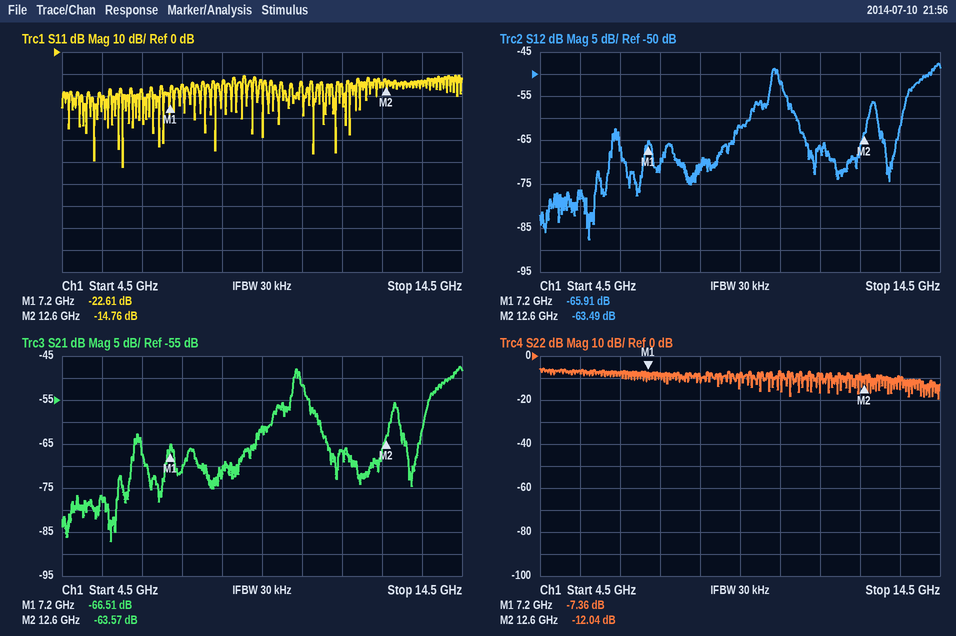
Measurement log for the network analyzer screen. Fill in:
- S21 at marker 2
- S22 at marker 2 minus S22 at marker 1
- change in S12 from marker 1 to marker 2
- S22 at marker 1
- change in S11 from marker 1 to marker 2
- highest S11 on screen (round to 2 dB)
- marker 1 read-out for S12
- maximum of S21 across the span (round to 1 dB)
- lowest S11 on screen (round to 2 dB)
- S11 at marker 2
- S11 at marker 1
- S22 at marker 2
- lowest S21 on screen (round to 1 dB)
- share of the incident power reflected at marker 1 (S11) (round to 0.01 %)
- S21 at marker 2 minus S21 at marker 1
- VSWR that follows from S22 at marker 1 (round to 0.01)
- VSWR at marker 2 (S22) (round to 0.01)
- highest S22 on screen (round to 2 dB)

-63.57 dB
-4.68 dB
2.42 dB
-7.36 dB
7.85 dB
-10 dB
-65.91 dB
-47 dB
-52 dB
-14.76 dB
-22.61 dB
-12.04 dB
-87 dB
0.55 %
2.94 dB
2.50
1.67
-6 dB
